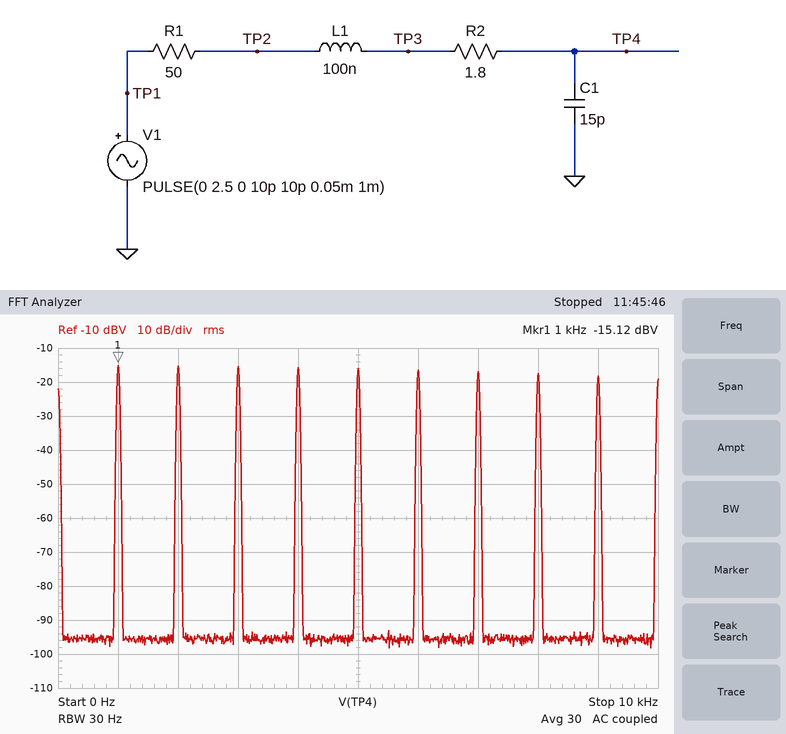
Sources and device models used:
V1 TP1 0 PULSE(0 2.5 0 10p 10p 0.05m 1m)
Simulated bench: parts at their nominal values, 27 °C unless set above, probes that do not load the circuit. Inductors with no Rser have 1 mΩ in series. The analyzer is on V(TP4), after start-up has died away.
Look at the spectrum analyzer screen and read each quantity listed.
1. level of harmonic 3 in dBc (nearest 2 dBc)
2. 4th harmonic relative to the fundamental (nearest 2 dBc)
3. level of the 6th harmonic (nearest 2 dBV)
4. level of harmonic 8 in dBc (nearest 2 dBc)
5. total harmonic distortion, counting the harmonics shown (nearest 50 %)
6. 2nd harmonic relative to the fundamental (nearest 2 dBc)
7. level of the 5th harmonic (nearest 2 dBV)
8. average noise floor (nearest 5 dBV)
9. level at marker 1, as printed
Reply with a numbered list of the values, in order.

1. 0 dBc
2. 0 dBc
3. -16 dBV
4. -2 dBc
5. 250 %
6. 0 dBc
7. -16 dBV
8. -95 dBV
9. -15.12 dBV
